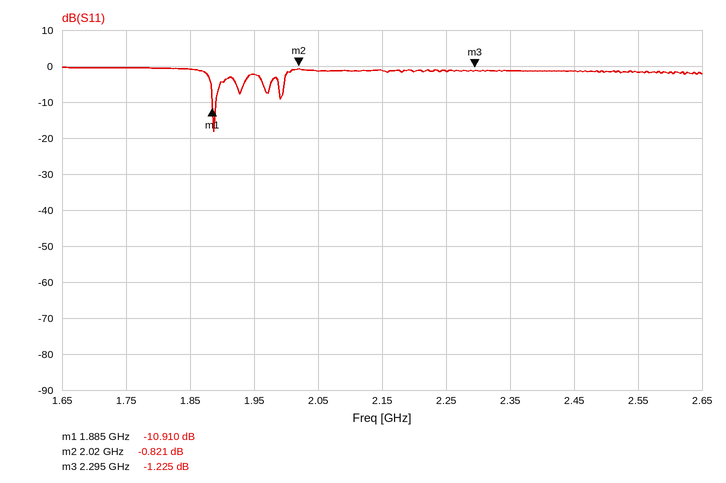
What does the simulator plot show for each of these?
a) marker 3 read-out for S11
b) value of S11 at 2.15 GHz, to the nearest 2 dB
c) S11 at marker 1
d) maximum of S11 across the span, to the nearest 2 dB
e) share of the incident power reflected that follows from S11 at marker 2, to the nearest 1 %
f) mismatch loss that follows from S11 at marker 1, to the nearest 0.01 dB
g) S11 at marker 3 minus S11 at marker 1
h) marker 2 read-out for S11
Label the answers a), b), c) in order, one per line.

a) -1.225 dB
b) -2 dB
c) -10.910 dB
d) 0 dB
e) 83 %
f) 0.37 dB
g) 9.685 dB
h) -0.821 dB
